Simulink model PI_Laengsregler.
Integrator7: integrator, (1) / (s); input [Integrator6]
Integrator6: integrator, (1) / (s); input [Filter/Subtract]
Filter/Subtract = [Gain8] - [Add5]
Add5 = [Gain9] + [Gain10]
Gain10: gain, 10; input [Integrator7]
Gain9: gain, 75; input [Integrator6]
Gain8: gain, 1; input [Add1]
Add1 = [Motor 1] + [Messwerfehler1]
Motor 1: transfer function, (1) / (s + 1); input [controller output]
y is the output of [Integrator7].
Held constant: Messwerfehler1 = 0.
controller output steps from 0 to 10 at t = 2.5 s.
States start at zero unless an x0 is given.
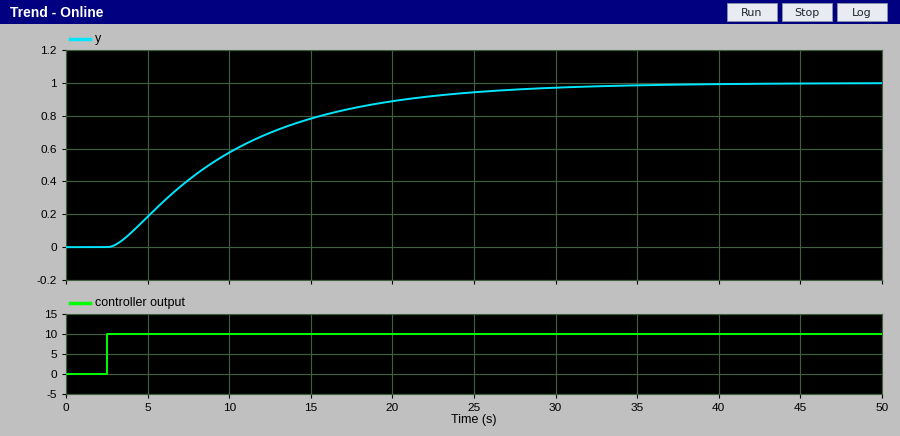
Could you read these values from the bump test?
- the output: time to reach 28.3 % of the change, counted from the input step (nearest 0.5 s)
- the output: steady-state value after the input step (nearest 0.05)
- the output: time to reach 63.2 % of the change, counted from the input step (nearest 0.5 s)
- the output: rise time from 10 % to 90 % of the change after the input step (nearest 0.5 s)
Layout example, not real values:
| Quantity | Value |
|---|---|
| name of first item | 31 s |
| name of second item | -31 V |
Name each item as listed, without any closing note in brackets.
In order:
| Quantity | Value |
|---|---|
| the output: time to reach 28.3 % of the change, counted from the input step | 3.5 s |
| the output: steady-state value after the input step | 1.00 |
| the output: time to reach 63.2 % of the change, counted from the input step | 8.5 s |
| the output: rise time from 10 % to 90 % of the change after the input step | 16.5 s |
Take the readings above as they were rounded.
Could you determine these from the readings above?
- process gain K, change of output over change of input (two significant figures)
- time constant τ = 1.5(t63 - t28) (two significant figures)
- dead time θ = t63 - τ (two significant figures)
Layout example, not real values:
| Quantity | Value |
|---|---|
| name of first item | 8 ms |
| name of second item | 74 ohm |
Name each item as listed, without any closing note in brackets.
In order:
| Quantity | Value |
|---|---|
| process gain K, change of output over change of input | 0.10 |
| time constant τ = 1.5(t63 - t28) | 7.5 s |
| dead time θ = t63 - τ | 1.0 s |
